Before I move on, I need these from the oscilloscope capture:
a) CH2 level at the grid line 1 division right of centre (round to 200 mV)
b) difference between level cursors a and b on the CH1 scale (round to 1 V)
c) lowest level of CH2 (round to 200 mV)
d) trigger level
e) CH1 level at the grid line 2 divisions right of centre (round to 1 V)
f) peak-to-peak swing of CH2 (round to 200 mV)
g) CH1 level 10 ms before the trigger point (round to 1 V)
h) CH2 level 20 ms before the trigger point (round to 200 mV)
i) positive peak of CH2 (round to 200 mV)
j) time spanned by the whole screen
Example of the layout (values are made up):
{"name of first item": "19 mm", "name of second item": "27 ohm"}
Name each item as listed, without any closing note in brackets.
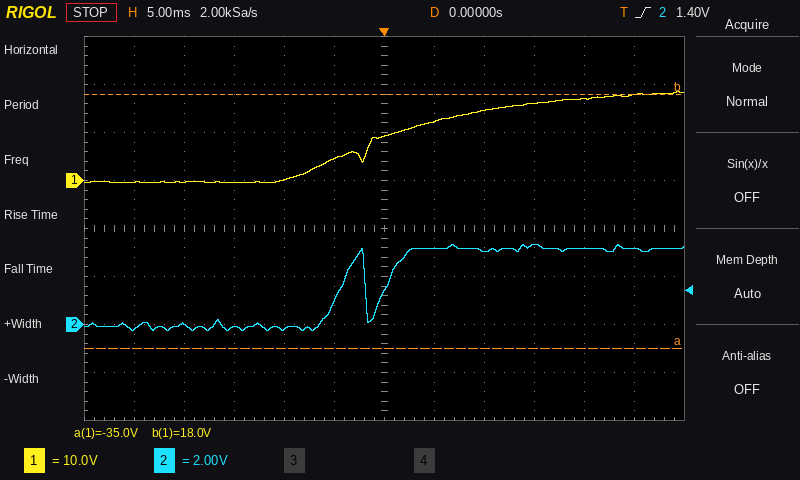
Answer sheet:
{"CH2 level at the grid line 1 division right of centre": "3.2 V", "difference between level cursors a and b on the CH1 scale": "53 V", "lowest level of CH2": "-200 mV", "trigger level": "1.40 V", "CH1 level at the grid line 2 divisions right of centre": "15 V", "peak-to-peak swing of CH2": "3.6 V", "CH1 level 10 ms before the trigger point": "0 V", "CH2 level 20 ms before the trigger point": "0.0 V", "positive peak of CH2": "3.4 V", "time spanned by the whole screen": "60 ms"}
